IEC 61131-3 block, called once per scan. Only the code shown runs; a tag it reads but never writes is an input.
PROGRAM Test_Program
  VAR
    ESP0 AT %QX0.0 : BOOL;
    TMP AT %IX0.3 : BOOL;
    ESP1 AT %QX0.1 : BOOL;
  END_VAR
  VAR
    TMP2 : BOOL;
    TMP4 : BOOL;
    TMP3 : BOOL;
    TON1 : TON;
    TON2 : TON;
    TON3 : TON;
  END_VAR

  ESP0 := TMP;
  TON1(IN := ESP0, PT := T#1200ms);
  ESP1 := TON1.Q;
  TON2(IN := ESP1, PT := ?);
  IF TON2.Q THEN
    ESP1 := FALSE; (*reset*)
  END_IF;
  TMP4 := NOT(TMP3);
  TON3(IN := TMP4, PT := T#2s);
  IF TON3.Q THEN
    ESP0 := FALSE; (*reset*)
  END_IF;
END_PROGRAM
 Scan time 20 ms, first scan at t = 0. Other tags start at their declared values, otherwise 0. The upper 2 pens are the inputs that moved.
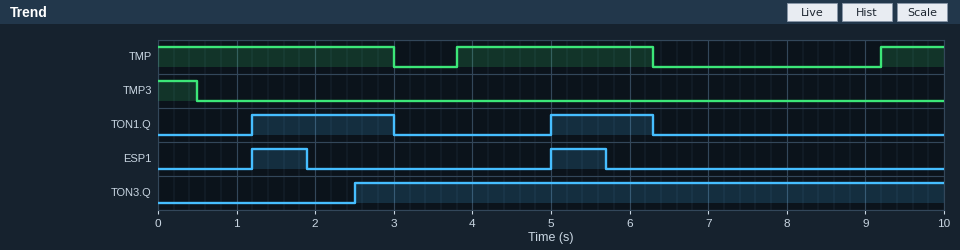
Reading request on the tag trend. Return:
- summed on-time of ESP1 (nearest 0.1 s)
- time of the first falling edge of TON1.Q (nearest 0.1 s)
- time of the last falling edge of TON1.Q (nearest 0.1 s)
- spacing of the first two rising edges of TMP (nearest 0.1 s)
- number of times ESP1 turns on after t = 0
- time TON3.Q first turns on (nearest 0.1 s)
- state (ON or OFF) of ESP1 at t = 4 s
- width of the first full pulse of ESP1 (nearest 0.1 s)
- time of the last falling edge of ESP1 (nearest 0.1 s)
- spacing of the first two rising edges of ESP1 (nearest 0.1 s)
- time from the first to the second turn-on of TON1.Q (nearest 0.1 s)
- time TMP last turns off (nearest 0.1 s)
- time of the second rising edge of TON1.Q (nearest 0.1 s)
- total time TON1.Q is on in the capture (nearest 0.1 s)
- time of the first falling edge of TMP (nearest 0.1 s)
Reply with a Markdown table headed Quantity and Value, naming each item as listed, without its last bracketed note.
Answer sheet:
| Quantity | Value |
|---|---|
| summed on-time of ESP1 | 1.4 s |
| time of the first falling edge of TON1.Q | 3.0 s |
| time of the last falling edge of TON1.Q | 6.3 s |
| spacing of the first two rising edges of TMP | 5.4 s |
| number of times ESP1 turns on after t = 0 | 2 |
| time TON3.Q first turns on | 2.5 s |
| state (ON or OFF) of ESP1 at t = 4 s | OFF |
| width of the first full pulse of ESP1 | 0.7 s |
| time of the last falling edge of ESP1 | 5.7 s |
| spacing of the first two rising edges of ESP1 | 3.8 s |
| time from the first to the second turn-on of TON1.Q | 3.8 s |
| time TMP last turns off | 6.3 s |
| time of the second rising edge of TON1.Q | 5.0 s |
| total time TON1.Q is on in the capture | 3.1 s |
| time of the first falling edge of TMP | 3.0 s |
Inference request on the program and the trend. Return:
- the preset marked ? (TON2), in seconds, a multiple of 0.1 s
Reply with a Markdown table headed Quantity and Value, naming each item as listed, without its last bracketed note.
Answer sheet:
| Quantity | Value |
|---|---|
| the preset marked ? (TON2), in seconds, a multiple of 0.1 s | 0.7 s |
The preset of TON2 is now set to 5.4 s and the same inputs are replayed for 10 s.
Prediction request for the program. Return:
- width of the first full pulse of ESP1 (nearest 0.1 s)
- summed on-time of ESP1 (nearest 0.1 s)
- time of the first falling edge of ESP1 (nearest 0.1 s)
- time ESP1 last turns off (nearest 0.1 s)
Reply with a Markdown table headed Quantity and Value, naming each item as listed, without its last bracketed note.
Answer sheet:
| Quantity | Value |
|---|---|
| width of the first full pulse of ESP1 | 1.8 s |
| summed on-time of ESP1 | 3.1 s |
| time of the first falling edge of ESP1 | 3.0 s |
| time ESP1 last turns off | 6.3 s |
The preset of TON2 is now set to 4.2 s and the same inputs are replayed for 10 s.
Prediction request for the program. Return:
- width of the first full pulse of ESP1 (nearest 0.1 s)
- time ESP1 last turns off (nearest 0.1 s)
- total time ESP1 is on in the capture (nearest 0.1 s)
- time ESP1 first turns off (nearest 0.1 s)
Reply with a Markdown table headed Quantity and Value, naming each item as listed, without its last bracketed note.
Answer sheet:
| Quantity | Value |
|---|---|
| width of the first full pulse of ESP1 | 1.8 s |
| time ESP1 last turns off | 6.3 s |
| total time ESP1 is on in the capture | 3.1 s |
| time ESP1 first turns off | 3.0 s |
